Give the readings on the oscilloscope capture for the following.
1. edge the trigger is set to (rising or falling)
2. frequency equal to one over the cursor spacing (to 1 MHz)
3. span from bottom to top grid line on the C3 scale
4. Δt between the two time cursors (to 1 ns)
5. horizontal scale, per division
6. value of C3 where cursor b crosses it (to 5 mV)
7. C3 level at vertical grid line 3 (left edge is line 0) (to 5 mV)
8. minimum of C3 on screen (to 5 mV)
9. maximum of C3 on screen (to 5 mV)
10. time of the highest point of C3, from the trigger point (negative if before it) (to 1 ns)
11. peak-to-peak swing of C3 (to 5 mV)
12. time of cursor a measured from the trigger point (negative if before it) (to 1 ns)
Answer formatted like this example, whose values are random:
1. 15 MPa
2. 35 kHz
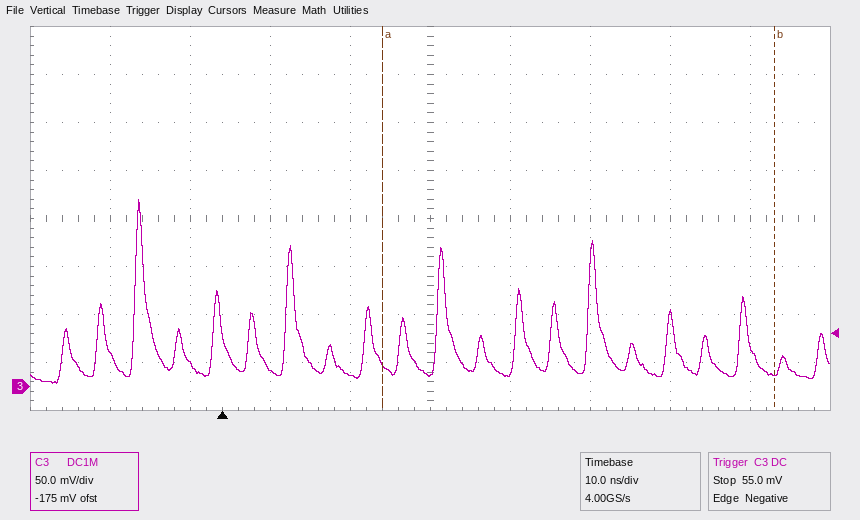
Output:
1. falling
2. 20 MHz
3. 400 mV
4. 49 ns
5. 10 ns
6. 15 mV
7. 20 mV
8. 5 mV
9. 195 mV
10. -10 ns
11. 190 mV
12. +20 ns
